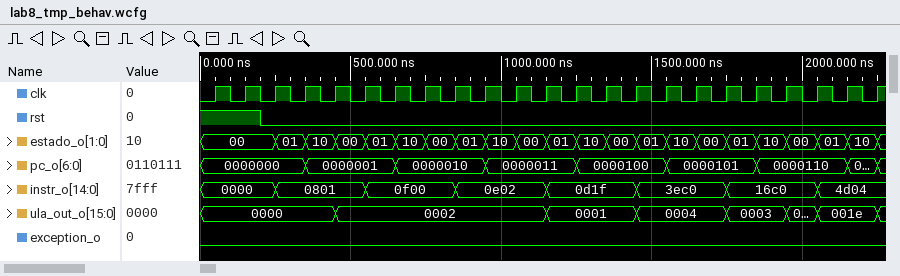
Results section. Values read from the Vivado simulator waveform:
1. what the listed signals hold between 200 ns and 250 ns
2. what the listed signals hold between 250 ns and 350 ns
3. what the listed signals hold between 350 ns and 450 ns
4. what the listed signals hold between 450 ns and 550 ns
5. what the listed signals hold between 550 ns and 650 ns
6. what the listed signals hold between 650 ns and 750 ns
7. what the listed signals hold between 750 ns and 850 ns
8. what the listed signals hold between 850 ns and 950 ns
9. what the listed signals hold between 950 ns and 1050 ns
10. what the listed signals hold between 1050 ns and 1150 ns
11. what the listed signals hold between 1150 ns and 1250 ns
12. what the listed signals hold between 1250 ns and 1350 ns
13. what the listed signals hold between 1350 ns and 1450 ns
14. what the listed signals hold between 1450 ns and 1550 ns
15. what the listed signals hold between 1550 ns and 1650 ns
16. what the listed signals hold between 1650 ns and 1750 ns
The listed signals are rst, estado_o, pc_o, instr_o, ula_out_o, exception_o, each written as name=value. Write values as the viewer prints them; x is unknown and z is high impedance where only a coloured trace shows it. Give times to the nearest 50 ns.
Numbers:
rst=0, estado_o=00, pc_o=0000000, instr_o=0000, ula_out_o=0000, exception_o=0
rst=0, estado_o=01, pc_o=0000000, instr_o=0801, ula_out_o=0000, exception_o=0
rst=0, estado_o=10, pc_o=0000001, instr_o=0801, ula_out_o=0000, exception_o=0
rst=0, estado_o=00, pc_o=0000001, instr_o=0801, ula_out_o=0002, exception_o=0
rst=0, estado_o=01, pc_o=0000001, instr_o=0f00, ula_out_o=0002, exception_o=0
rst=0, estado_o=10, pc_o=0000010, instr_o=0f00, ula_out_o=0002, exception_o=0
rst=0, estado_o=00, pc_o=0000010, instr_o=0f00, ula_out_o=0002, exception_o=0
rst=0, estado_o=01, pc_o=0000010, instr_o=0e02, ula_out_o=0002, exception_o=0
rst=0, estado_o=10, pc_o=0000011, instr_o=0e02, ula_out_o=0002, exception_o=0
rst=0, estado_o=00, pc_o=0000011, instr_o=0e02, ula_out_o=0002, exception_o=0
rst=0, estado_o=01, pc_o=0000011, instr_o=0d1f, ula_out_o=0001, exception_o=0
rst=0, estado_o=10, pc_o=0000100, instr_o=0d1f, ula_out_o=0001, exception_o=0
rst=0, estado_o=00, pc_o=0000100, instr_o=0d1f, ula_out_o=0001, exception_o=0
rst=0, estado_o=01, pc_o=0000100, instr_o=3ec0, ula_out_o=0004, exception_o=0
rst=0, estado_o=10, pc_o=0000101, instr_o=3ec0, ula_out_o=0004, exception_o=0
rst=0, estado_o=00, pc_o=0000101, instr_o=3ec0, ula_out_o=0004, exception_o=0
